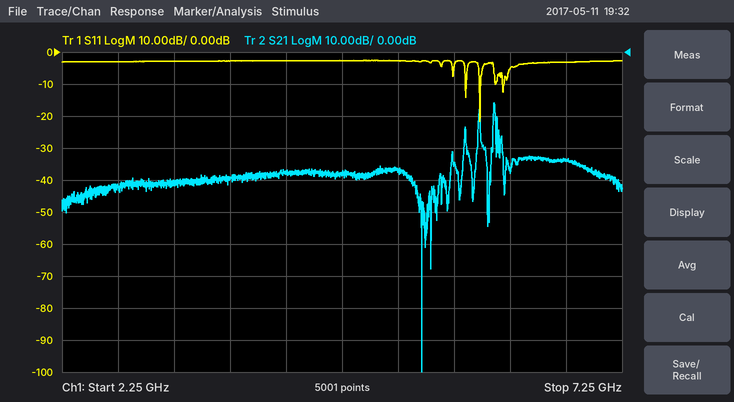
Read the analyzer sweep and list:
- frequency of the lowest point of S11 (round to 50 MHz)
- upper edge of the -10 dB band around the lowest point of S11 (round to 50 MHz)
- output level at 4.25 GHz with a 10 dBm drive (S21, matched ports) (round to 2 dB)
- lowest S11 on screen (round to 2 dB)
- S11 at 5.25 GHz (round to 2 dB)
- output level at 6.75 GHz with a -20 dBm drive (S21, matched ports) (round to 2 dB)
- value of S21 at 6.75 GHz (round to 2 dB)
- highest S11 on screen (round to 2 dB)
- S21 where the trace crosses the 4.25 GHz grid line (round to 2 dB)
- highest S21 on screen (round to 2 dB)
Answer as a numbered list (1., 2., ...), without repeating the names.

1. 6.00 GHz
2. 6.00 GHz
3. -28 dBm
4. -22 dB
5. -2 dB
6. -54 dBm
7. -34 dB
8. -2 dB
9. -38 dB
10. -16 dB
